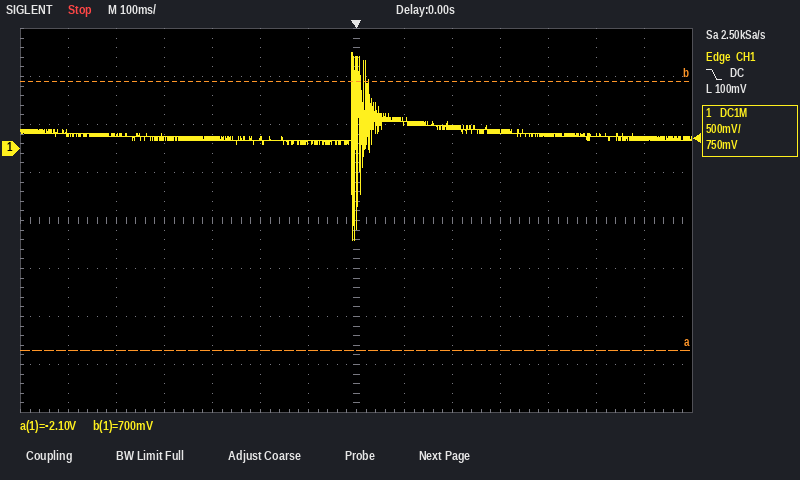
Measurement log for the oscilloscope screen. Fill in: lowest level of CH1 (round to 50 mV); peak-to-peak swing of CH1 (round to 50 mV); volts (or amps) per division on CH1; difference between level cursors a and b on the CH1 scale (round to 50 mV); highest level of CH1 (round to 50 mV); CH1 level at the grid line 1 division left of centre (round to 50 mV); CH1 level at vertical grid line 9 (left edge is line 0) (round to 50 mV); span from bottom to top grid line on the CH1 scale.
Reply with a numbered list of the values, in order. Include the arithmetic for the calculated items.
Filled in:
1. -950 mV
2. 1.00 V − (-950 mV) = 1.95 V
3. 500 mV
4. 2.80 V
5. 1.00 V
6. 50 mV
7. 200 mV
8. 4 V
